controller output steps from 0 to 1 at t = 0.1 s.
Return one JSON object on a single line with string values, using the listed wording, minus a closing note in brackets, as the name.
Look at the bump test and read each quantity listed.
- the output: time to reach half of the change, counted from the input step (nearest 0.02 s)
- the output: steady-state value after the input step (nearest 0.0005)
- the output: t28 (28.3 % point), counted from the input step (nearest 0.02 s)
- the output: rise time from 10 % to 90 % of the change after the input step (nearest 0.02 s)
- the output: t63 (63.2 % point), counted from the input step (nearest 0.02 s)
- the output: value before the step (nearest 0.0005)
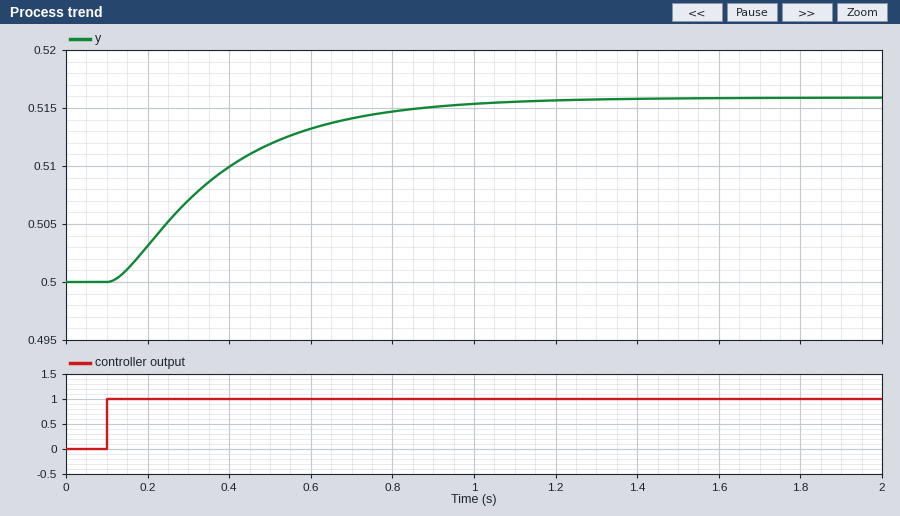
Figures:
{"the output: time to reach half of the change, counted from the input step": "0.22 s", "the output: steady-state value after the input step": "0.5160", "the output: t28 (28.3 % point), counted from the input step": "0.14 s", "the output: rise time from 10 % to 90 % of the change after the input step": "0.56 s", "the output: t63 (63.2 % point), counted from the input step": "0.30 s", "the output: value before the step": "0.5000"}
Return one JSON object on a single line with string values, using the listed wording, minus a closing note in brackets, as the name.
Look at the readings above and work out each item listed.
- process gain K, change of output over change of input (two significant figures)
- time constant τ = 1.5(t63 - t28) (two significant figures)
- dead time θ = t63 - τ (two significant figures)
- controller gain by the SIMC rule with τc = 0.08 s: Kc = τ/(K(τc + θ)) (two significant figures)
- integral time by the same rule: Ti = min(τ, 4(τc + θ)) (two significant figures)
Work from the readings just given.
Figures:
{"process gain K, change of output over change of input": "0.016", "time constant τ = 1.5(t63 - t28)": "0.24 s", "dead time θ = t63 - τ": "0.060 s", "controller gain by the SIMC rule with τc = 0.08 s: Kc = τ/(K(τc + θ))": "110", "integral time by the same rule: Ti = min(τ, 4(τc + θ))": "0.24 s"}
